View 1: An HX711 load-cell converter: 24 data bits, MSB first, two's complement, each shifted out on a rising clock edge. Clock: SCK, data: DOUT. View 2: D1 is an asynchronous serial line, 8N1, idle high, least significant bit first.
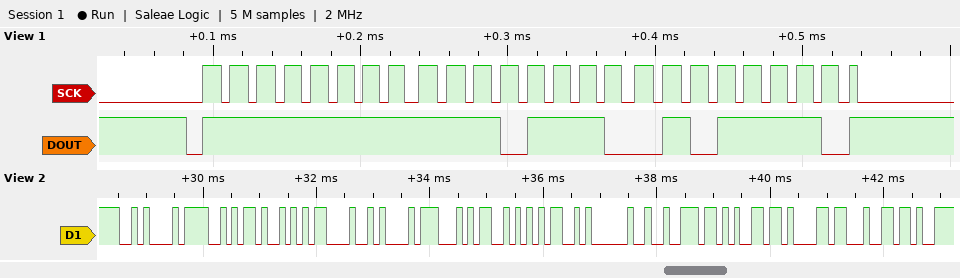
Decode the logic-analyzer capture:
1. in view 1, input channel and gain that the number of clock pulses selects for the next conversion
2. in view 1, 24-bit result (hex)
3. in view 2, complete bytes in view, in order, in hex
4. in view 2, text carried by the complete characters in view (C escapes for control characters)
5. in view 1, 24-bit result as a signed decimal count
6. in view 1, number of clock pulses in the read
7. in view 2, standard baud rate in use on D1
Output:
channel A, gain 128
0xFFEE5E
0A 4F 4B 0D 0A 47 53 4D 20 72 65 61 64
"\nOK\r\nGSM read"
-4514
25
9600 baud
